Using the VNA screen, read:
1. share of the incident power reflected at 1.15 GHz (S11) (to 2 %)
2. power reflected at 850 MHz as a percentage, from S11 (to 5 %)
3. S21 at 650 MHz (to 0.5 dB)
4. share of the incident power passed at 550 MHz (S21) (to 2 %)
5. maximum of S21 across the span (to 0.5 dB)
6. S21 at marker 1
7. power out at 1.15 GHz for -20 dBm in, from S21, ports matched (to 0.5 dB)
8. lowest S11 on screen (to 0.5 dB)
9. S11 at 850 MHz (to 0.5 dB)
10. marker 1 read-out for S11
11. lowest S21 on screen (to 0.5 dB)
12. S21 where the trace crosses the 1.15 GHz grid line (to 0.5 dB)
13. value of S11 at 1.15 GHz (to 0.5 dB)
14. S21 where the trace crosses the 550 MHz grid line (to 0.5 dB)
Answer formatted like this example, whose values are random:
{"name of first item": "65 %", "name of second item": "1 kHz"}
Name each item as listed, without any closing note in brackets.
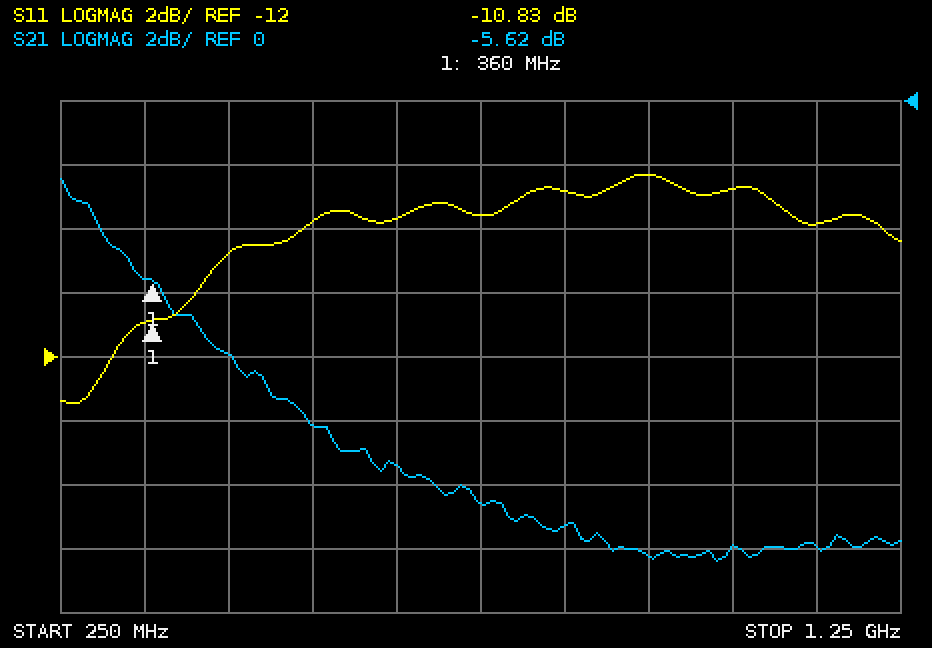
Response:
{"share of the incident power reflected at 1.15 GHz (S11)": "16 %", "power reflected at 850 MHz as a percentage, from S11": "20 %", "S21 at 650 MHz": "-11.5 dB", "share of the incident power passed at 550 MHz (S21)": "10 %", "maximum of S21 across the span": "-2.5 dB", "S21 at marker 1": "-5.62 dB", "power out at 1.15 GHz for -20 dBm in, from S21, ports matched": "-34.0 dBm", "lowest S11 on screen": "-13.5 dB", "S11 at 850 MHz": "-7.0 dB", "marker 1 read-out for S11": "-10.83 dB", "lowest S21 on screen": "-14.5 dB", "S21 where the trace crosses the 1.15 GHz grid line": "-14.0 dB", "value of S11 at 1.15 GHz": "-8.0 dB", "S21 where the trace crosses the 550 MHz grid line": "-10.0 dB"}
